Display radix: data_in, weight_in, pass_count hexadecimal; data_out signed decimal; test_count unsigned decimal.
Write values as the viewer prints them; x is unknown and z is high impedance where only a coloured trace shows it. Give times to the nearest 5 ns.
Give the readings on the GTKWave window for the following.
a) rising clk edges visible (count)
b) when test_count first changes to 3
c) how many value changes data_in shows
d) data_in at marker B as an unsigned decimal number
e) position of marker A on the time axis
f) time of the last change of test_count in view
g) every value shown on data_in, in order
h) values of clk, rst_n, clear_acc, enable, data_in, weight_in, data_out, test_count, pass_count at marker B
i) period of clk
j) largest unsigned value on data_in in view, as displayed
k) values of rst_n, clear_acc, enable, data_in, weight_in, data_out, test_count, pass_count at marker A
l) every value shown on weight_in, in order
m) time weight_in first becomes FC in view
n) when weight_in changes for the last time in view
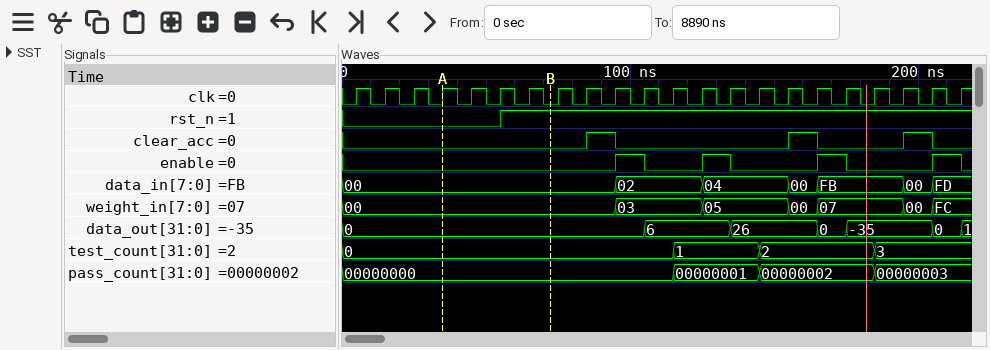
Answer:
22
185 ns
6
0
35 ns
185 ns
00, 02, 04, 00, FB, 00, FD
clk=0, rst_n=1, clear_acc=0, enable=0, data_in=00, weight_in=00, data_out=0, test_count=0, pass_count=00000000
10 ns
FD
rst_n=0, clear_acc=0, enable=0, data_in=00, weight_in=00, data_out=0, test_count=0, pass_count=00000000
00, 03, 05, 00, 07, 00, FC
205 ns
205 ns
